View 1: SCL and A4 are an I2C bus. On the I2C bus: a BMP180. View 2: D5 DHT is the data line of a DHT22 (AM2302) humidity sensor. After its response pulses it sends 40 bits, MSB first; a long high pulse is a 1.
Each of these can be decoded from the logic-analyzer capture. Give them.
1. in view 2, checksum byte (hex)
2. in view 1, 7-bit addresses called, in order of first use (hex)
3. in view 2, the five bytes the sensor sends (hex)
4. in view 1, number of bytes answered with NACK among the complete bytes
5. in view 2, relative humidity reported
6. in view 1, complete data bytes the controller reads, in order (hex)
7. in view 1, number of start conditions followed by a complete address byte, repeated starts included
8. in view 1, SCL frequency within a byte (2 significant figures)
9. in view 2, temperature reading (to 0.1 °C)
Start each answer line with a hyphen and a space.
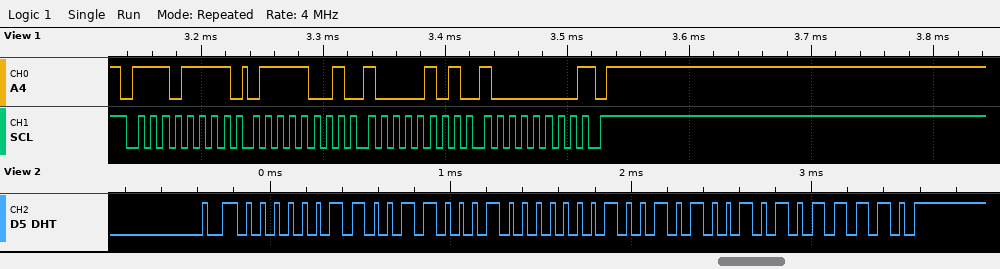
- 0x5E
- 0x77
- 03 31 01 29 5E
- 1
- 81.7 %
- 79 85 80
- 1
- 100 kHz
- 29.7 °C
